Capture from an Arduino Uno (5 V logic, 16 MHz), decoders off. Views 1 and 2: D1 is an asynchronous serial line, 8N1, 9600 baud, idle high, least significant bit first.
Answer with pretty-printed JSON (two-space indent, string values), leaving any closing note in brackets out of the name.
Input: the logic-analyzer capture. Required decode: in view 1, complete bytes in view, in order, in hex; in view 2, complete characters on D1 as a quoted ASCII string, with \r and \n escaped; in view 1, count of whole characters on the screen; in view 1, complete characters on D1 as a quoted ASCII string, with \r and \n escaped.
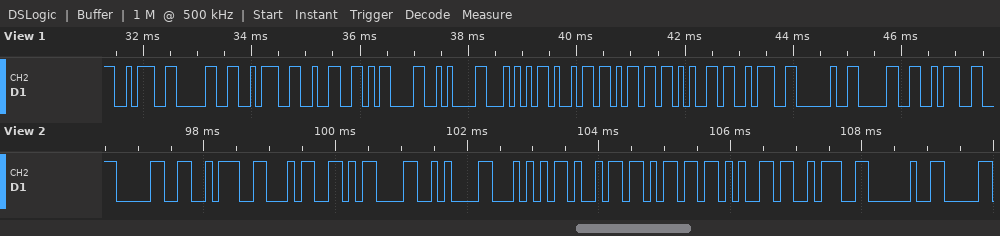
{
  "in view 1, complete bytes in view, in order, in hex": "0x3A 0x30 0x3A 0x32 0x0D 0x0A 0x54 0x69 0x6D 0x65 0x3A 0x20 0x30 0x3A",
  "in view 2, complete characters on D1 as a quoted ASCII string, with \\r and \\n escaped": "\"0:4\\r\\nTime: \"",
  "in view 1, count of whole characters on the screen": "14",
  "in view 1, complete characters on D1 as a quoted ASCII string, with \\r and \\n escaped": "\":0:2\\r\\nTime: 0:\""
}
